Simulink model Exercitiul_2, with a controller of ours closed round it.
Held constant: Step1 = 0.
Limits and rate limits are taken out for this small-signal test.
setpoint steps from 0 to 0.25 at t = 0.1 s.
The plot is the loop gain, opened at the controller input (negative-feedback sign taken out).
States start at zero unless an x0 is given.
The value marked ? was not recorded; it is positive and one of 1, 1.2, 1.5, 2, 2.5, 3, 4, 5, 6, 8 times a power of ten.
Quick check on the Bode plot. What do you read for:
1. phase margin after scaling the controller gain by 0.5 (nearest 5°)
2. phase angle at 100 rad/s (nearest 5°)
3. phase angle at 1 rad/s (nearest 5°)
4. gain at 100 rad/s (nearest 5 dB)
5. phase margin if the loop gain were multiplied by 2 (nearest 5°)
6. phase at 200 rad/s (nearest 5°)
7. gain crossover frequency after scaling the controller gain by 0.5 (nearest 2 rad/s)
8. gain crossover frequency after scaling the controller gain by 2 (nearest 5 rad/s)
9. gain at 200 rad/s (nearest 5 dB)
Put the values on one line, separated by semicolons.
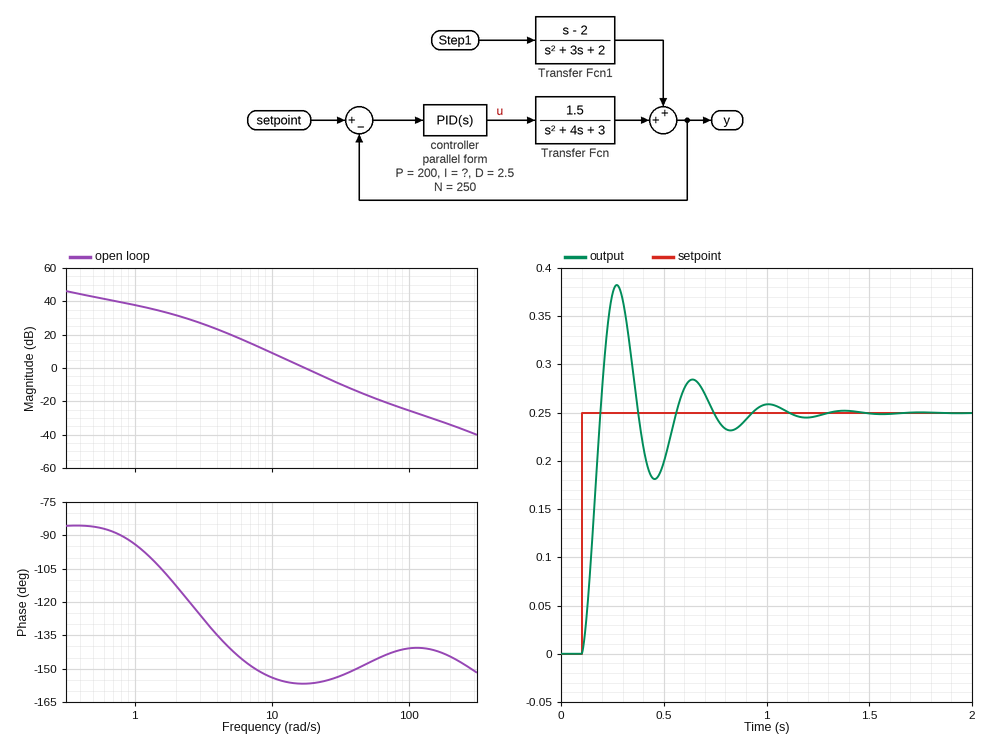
25°; -140°; -95°; -25 dB; 25°; -145°; 12 rad/s; 25 rad/s; -35 dB
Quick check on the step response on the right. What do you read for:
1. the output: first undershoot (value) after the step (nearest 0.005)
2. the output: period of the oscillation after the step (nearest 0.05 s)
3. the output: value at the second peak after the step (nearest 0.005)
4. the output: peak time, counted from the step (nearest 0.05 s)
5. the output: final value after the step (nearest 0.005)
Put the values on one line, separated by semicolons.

0.180; 0.35 s; 0.285; 0.15 s; 0.250
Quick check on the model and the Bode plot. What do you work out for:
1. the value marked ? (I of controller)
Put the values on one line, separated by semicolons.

120
